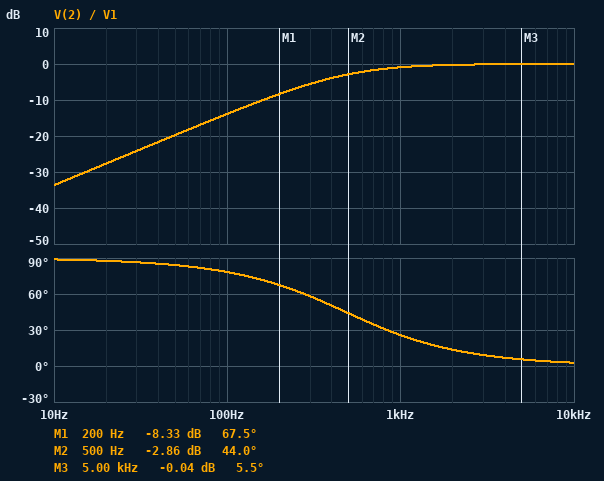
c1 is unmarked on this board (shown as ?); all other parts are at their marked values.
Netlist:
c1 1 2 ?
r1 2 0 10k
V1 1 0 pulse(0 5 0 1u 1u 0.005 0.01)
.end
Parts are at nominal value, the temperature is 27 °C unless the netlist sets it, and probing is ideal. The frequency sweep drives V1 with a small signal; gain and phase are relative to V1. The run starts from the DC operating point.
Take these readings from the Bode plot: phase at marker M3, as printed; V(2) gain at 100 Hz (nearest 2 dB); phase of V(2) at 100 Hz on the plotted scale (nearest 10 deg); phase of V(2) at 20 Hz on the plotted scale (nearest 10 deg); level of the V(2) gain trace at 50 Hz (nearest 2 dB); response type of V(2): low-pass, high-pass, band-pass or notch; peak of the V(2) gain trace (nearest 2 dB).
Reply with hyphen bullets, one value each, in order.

- 5.5 deg
- -14 dB
- 80 deg
- 90 deg
- -20 dB
- high-pass
- 0 dB
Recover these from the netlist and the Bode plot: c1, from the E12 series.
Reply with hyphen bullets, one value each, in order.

- 33 nF
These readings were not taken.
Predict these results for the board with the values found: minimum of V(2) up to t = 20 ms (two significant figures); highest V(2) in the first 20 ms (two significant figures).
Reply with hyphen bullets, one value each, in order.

- -5.0 V
- 5.0 V
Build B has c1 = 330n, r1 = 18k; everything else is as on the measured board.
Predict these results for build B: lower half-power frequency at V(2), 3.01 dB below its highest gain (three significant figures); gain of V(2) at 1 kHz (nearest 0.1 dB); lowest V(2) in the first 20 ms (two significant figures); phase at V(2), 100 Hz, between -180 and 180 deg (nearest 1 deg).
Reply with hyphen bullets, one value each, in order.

- 26.8 Hz
- 0 dB
- -3.4 V
- 15 deg
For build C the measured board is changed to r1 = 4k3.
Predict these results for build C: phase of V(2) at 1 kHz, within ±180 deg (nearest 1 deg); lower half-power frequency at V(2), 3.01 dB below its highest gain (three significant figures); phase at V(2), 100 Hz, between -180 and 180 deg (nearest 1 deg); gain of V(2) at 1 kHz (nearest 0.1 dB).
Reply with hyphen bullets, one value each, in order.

- 48 deg
- 1.12 kHz
- 85 deg
- -3.5 dB
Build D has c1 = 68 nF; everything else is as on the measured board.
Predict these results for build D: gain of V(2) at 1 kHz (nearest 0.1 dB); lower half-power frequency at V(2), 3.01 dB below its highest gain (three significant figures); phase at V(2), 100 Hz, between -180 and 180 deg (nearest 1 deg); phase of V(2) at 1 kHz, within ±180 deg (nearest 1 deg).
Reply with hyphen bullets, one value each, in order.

- -0.2 dB
- 234 Hz
- 67 deg
- 13 deg
